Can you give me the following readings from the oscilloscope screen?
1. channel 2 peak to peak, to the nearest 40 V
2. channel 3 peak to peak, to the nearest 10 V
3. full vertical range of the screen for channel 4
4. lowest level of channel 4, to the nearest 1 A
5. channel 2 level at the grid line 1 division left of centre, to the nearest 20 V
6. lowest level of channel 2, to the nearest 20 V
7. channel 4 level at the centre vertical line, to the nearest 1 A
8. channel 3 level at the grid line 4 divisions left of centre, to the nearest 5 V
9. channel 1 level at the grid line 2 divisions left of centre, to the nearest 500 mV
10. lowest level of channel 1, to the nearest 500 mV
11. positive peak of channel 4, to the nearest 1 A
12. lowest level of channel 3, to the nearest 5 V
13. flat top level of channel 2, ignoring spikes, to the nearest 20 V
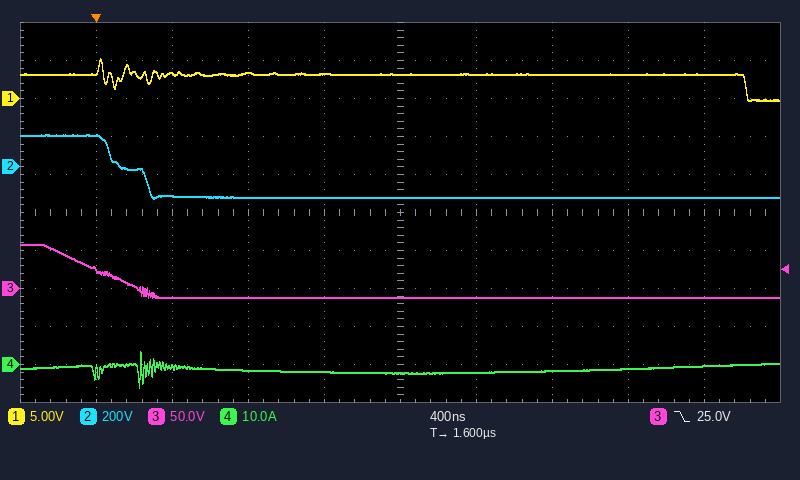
320 V
70 V
100 A
-6 A
-160 V
-160 V
-2 A
25 V
3.5 V
-500 mV
3 A
-10 V
160 V
